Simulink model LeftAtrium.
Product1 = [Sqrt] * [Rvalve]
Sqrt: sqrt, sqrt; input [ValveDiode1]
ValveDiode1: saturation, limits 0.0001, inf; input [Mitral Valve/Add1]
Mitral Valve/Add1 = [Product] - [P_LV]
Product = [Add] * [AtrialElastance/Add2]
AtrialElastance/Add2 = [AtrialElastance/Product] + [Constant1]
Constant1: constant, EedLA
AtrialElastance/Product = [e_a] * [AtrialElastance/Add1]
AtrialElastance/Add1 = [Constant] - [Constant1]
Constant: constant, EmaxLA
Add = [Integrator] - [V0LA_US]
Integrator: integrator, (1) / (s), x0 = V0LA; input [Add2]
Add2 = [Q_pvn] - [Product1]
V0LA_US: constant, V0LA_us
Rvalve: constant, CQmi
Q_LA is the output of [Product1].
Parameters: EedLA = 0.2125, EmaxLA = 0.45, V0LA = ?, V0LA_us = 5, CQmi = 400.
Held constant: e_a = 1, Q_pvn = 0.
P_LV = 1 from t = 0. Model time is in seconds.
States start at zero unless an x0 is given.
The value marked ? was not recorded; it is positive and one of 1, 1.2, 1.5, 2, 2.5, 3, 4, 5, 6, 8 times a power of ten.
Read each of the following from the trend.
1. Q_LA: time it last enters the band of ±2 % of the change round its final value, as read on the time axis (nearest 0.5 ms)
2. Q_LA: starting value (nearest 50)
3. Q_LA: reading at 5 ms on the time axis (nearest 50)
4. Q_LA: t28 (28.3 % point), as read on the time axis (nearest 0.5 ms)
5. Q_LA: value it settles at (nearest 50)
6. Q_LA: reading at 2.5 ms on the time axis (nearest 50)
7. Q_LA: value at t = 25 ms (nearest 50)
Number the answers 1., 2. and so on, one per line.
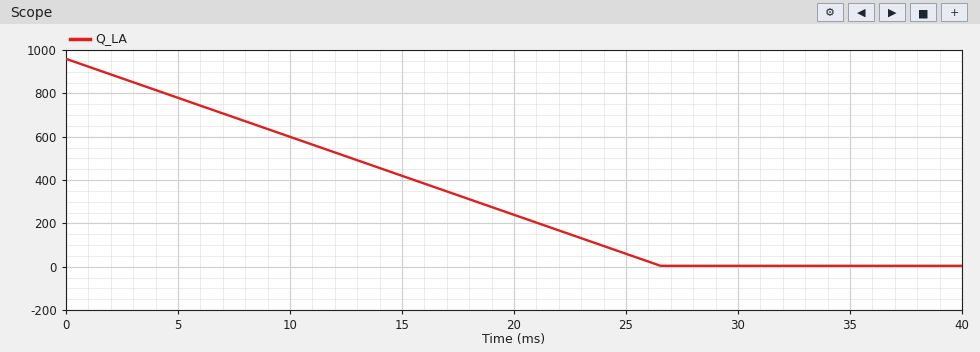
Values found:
1. 26.0 ms
2. 950
3. 800
4. 7.5 ms
5. 0
6. 850
7. 50
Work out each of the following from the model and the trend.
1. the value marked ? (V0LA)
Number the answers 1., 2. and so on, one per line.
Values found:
1. 20
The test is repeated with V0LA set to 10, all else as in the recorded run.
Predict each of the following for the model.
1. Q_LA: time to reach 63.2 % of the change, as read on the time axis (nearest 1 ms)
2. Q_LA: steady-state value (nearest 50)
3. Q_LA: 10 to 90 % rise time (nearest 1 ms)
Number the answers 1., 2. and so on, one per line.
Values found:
1. 8 ms
2. 0
3. 10 ms
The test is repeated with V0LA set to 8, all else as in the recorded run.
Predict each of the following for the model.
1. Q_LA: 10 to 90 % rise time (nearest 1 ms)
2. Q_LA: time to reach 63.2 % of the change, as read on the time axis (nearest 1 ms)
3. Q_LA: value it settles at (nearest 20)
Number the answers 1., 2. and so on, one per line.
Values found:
1. 5 ms
2. 4 ms
3. 0
